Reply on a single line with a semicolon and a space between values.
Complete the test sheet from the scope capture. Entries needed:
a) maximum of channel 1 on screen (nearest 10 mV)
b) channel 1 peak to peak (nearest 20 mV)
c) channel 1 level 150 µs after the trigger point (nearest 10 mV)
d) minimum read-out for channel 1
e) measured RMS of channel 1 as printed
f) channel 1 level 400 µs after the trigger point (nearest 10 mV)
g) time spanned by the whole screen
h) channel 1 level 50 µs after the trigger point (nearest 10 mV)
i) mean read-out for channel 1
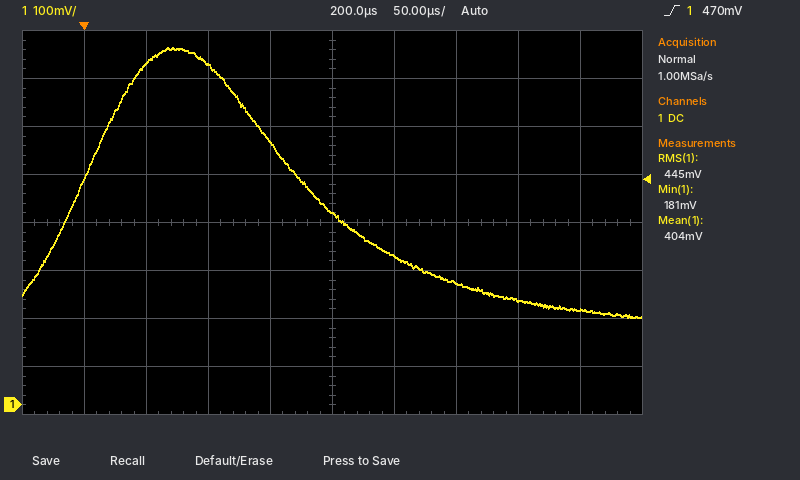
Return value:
740 mV; 560 mV; 550 mV; 181 mV; 445 mV; 200 mV; 500 µs; 710 mV; 404 mV
